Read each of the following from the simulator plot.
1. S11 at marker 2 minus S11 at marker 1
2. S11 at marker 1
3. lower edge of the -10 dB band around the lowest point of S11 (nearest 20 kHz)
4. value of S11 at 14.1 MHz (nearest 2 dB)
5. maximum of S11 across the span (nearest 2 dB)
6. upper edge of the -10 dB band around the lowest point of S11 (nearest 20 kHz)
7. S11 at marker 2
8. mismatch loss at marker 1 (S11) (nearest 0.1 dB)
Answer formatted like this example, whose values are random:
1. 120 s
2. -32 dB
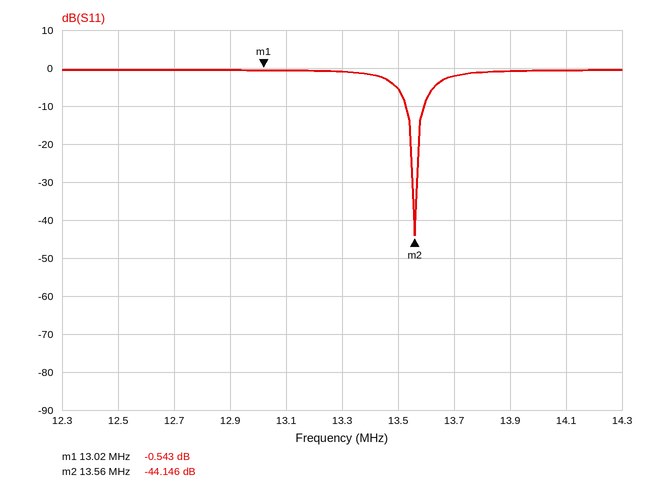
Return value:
1. -43.603 dB
2. -0.543 dB
3. 13.52 MHz
4. 0 dB
5. 0 dB
6. 13.60 MHz
7. -44.146 dB
8. 9.3 dB
